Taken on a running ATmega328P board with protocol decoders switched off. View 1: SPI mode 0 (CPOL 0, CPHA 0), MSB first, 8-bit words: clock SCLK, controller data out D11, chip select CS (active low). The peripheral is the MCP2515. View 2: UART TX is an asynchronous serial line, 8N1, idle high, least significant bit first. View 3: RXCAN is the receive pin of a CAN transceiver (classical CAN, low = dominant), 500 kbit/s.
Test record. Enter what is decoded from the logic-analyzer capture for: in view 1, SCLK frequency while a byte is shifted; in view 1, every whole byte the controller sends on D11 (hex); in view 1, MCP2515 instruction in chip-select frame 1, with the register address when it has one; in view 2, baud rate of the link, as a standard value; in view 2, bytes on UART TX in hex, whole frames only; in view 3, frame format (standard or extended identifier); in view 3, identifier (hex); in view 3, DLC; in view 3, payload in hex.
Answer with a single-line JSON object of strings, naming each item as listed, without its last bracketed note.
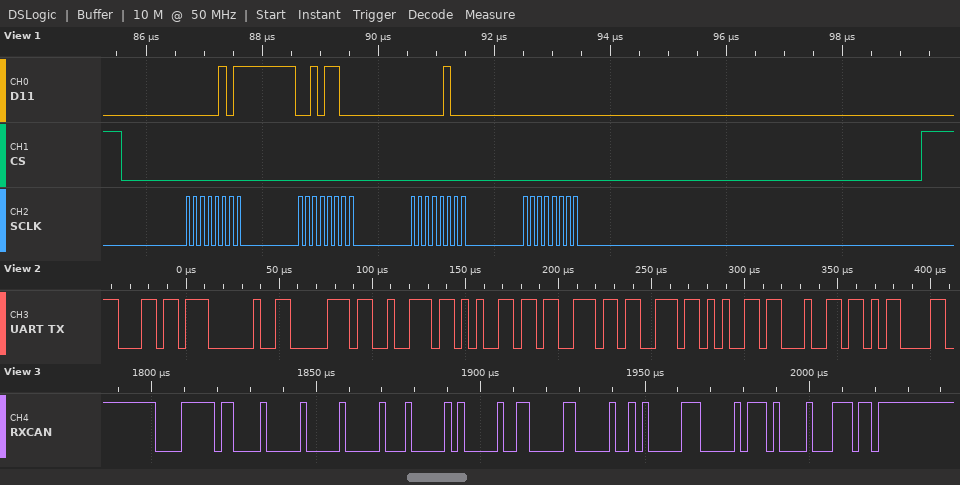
{"in view 1, SCLK frequency while a byte is shifted": "8 MHz", "in view 1, every whole byte the controller sends on D11": "05 2C 04 00", "in view 1, MCP2515 instruction in chip-select frame 1, with the register address when it has one": "BIT MODIFY 0x2C", "in view 2, baud rate of the link, as a standard value": "250000 baud", "in view 2, bytes on UART TX in hex, whole frames only": "6C 20 70 72 65 73 73 65 64 0D", "in view 3, frame format": "standard", "in view 3, identifier": "0x0FE", "in view 3, DLC": "8", "in view 3, payload in hex": "00 01 02 03 04 05 06 07"}
